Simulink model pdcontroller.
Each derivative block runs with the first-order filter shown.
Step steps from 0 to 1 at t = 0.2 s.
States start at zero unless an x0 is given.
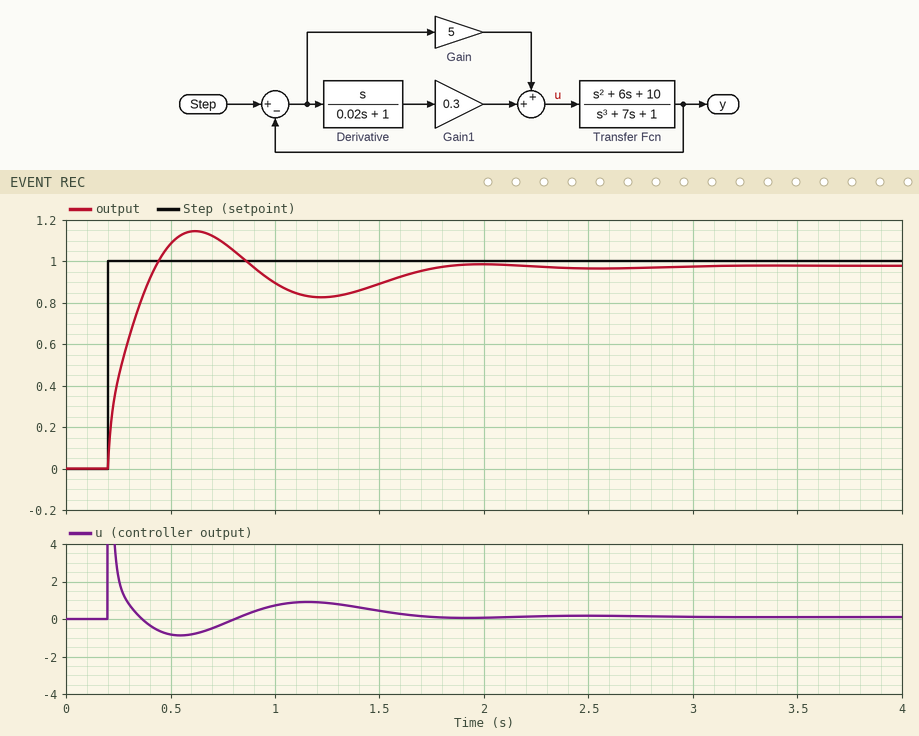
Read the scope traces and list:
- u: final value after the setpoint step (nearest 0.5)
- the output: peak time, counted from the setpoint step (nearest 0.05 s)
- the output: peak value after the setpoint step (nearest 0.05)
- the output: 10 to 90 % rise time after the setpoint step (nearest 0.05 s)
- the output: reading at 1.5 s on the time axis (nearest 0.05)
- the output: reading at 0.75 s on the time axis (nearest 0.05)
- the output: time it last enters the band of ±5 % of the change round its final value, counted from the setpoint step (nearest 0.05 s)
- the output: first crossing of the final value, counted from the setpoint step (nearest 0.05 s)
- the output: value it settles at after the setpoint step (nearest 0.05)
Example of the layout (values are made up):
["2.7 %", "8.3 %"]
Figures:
["0.0", "0.40 s", "1.15", "0.20 s", "0.90", "1.10", "1.40 s", "0.25 s", "1.00"]
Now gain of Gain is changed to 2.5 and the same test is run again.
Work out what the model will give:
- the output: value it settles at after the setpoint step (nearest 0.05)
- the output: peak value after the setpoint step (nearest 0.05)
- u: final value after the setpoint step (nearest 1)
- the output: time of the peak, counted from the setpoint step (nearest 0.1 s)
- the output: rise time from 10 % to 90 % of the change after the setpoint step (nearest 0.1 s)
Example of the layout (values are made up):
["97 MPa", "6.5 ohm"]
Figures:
["0.95", "1.10", "0", "0.5 s", "0.3 s"]
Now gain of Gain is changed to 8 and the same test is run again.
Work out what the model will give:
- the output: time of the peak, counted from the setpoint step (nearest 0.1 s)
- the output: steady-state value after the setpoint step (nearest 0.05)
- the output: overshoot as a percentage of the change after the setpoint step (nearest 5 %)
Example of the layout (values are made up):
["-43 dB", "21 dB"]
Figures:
["0.3 s", "1.00", "15 %"]
